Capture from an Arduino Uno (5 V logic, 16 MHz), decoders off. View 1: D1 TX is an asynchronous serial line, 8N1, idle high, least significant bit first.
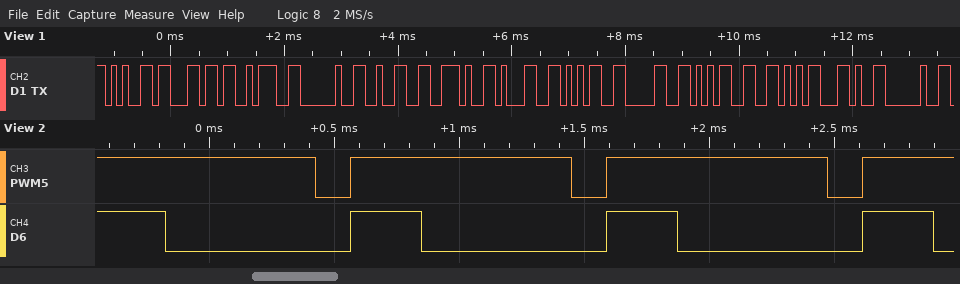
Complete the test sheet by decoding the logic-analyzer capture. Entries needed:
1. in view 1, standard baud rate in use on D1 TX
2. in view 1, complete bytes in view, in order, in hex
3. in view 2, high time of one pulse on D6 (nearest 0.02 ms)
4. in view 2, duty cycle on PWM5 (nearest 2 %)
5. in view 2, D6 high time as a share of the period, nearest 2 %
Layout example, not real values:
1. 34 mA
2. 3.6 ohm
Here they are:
1. 9600 baud
2. 65 6C 3A 20 32 2E 31 35 30 35 56 2C 20
3. 0.28 ms
4. 86 %
5. 28 %
